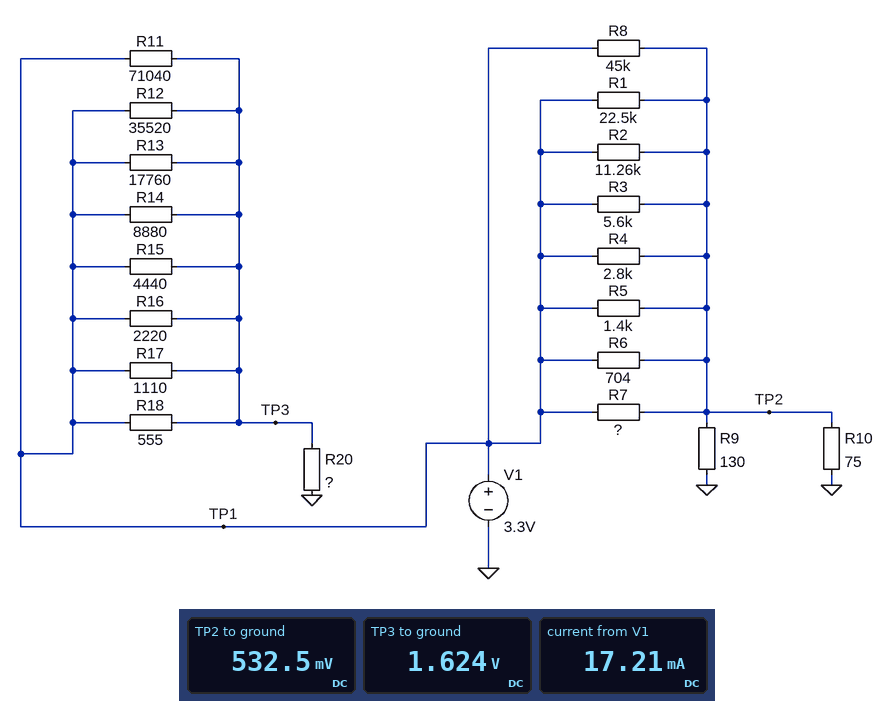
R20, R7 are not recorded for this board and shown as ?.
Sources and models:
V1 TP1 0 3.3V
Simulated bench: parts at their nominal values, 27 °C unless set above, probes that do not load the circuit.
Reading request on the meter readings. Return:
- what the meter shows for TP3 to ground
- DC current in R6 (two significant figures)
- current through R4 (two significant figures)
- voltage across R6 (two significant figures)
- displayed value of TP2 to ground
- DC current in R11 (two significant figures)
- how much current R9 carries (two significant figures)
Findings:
1.624 V
3.9 mA
990 µA
2.8 V
532.5 mV
24 µA
4.1 mA
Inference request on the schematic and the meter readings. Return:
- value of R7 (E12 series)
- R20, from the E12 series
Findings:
820 Ω
270 Ω
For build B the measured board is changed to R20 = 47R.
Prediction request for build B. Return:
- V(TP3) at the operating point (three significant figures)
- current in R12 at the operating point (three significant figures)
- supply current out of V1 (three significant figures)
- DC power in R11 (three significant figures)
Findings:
476 mV
79.5 µA
21.3 mA
112 µW
